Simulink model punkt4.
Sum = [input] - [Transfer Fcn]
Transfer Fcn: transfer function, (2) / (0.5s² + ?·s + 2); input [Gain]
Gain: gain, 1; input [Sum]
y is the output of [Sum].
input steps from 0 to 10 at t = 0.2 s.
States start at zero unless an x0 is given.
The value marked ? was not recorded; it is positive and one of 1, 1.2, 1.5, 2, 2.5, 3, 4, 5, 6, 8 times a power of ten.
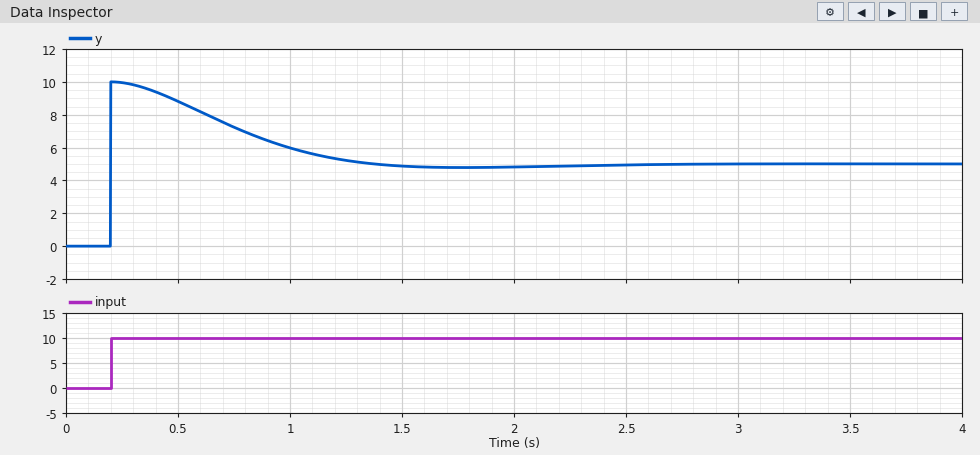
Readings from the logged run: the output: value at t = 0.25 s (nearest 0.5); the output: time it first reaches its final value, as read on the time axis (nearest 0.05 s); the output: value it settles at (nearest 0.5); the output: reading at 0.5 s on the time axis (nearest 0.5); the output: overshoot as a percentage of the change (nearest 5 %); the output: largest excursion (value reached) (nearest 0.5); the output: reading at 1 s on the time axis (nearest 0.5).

10.0
0.20 s
5.0
9.0
100 %
10.0
6.0
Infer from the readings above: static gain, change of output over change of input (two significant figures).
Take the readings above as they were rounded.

0.50
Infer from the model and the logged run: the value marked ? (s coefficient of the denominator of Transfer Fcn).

2
